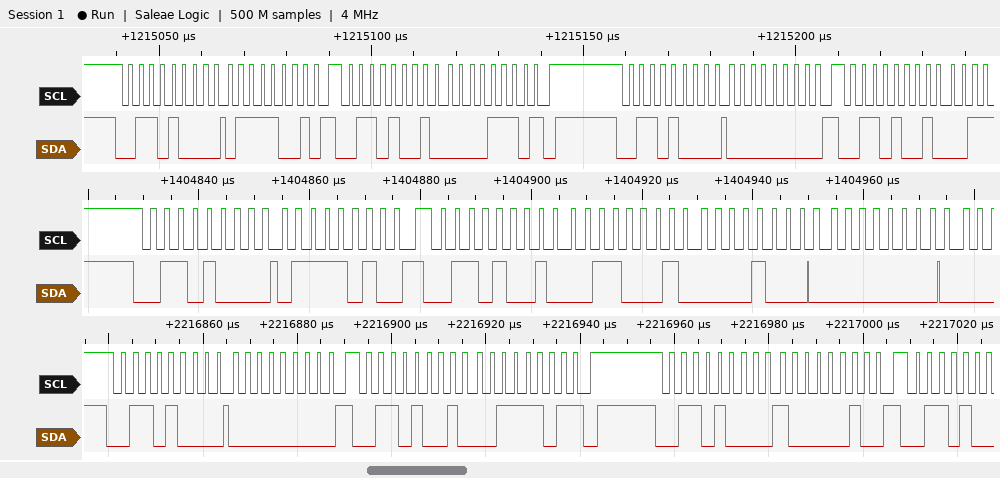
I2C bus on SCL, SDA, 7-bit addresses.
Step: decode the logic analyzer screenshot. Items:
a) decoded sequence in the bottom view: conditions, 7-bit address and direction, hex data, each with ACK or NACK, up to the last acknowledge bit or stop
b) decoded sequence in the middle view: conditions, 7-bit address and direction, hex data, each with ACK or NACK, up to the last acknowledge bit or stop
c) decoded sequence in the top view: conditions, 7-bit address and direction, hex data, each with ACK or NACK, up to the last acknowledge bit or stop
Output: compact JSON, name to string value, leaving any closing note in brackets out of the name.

{"decoded sequence in the bottom view: conditions, 7-bit address and direction, hex data, each with ACK or NACK, up to the last acknowledge bit or stop": "start, address 34 write ACK, 00 ACK, repeated start, address 34 read ACK, 3D NACK, stop, start, address 34 write ACK, 82 ACK", "decoded sequence in the middle view: conditions, 7-bit address and direction, hex data, each with ACK or NACK, up to the last acknowledge bit or stop": "start, address 34 write ACK, 7A ACK, repeated start, address 34 read ACK, 31 ACK, 08 ACK, 00 ACK", "decoded sequence in the top view: conditions, 7-bit address and direction, hex data, each with ACK or NACK, up to the last acknowledge bit or stop": "start, address 34 write ACK, 79 ACK, repeated start, address 34 read ACK, 0E NACK, stop, start, address 34 write ACK, 00 ACK, repeated start, address 34 read ACK"}
